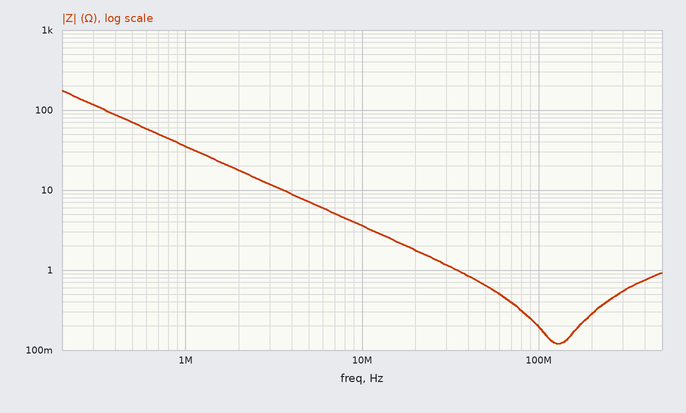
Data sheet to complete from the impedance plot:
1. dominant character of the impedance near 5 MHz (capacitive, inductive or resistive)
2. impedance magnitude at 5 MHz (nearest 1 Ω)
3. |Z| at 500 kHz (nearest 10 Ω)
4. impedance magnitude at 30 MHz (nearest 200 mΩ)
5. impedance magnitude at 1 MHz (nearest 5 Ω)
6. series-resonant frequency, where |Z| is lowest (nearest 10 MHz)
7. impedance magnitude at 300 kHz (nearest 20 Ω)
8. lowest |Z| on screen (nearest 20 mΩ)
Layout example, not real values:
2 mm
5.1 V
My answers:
capacitive
7 Ω
70 Ω
1.2 Ω
35 Ω
130 MHz
120 Ω
120 mΩ
